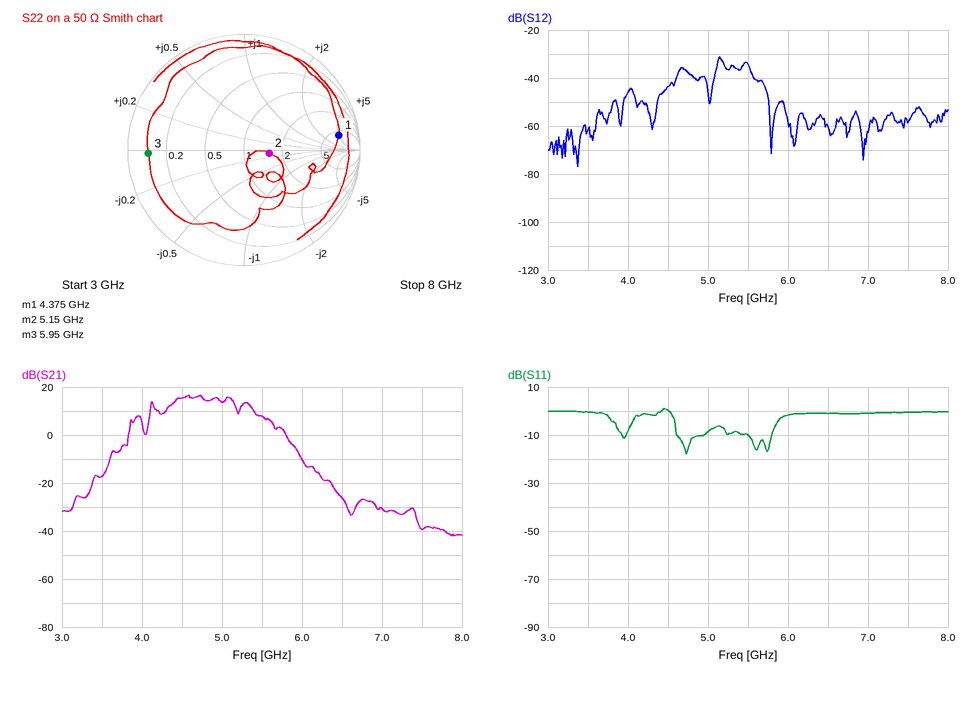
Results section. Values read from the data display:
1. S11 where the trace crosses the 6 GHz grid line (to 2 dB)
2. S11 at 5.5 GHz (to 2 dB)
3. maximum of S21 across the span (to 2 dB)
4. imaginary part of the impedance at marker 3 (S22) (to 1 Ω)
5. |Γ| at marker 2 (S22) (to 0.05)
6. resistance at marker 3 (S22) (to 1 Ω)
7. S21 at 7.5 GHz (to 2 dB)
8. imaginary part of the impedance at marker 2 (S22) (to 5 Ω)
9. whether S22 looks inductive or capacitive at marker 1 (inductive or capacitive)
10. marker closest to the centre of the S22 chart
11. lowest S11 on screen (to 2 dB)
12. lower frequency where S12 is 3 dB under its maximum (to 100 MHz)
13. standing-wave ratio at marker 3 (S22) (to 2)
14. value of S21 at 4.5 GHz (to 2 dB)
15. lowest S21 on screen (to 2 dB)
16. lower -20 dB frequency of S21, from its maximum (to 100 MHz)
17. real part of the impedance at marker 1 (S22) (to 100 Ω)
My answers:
-2 dB
-10 dB
16 dB
-1 Ω
0.20
5 Ω
-40 dB
-5 Ω
inductive
marker 2
-18 dB
5.1 GHz
10
16 dB
-42 dB
3.8 GHz
300 Ω
